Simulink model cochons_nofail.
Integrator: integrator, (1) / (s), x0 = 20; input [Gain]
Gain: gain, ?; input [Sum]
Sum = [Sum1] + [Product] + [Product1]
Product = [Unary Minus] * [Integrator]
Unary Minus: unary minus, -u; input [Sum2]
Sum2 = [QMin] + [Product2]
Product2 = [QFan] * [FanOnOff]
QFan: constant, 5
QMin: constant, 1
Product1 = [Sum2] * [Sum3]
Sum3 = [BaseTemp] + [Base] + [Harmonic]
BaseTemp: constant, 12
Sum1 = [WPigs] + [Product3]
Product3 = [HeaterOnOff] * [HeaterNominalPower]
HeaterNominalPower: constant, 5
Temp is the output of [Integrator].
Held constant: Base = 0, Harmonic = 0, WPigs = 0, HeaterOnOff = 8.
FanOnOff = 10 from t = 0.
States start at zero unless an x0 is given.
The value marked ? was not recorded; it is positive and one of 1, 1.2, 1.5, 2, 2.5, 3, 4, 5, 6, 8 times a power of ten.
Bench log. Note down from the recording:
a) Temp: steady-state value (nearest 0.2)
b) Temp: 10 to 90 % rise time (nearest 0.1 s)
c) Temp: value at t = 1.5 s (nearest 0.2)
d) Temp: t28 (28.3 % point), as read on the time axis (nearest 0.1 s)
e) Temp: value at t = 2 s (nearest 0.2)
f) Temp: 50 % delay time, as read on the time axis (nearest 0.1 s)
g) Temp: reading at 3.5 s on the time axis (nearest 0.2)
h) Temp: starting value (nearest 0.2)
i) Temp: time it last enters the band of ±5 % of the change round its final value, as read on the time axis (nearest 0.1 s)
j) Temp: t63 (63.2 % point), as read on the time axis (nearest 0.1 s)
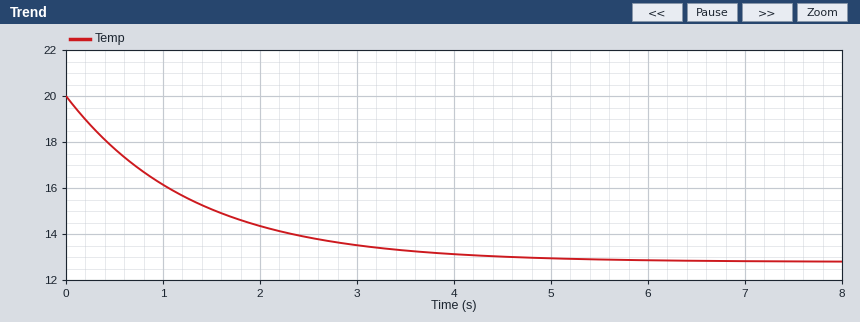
12.8
2.9 s
15.0
0.4 s
14.4
0.9 s
13.2
20.0
3.9 s
1.3 s
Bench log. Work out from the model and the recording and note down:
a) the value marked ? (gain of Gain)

0.015
